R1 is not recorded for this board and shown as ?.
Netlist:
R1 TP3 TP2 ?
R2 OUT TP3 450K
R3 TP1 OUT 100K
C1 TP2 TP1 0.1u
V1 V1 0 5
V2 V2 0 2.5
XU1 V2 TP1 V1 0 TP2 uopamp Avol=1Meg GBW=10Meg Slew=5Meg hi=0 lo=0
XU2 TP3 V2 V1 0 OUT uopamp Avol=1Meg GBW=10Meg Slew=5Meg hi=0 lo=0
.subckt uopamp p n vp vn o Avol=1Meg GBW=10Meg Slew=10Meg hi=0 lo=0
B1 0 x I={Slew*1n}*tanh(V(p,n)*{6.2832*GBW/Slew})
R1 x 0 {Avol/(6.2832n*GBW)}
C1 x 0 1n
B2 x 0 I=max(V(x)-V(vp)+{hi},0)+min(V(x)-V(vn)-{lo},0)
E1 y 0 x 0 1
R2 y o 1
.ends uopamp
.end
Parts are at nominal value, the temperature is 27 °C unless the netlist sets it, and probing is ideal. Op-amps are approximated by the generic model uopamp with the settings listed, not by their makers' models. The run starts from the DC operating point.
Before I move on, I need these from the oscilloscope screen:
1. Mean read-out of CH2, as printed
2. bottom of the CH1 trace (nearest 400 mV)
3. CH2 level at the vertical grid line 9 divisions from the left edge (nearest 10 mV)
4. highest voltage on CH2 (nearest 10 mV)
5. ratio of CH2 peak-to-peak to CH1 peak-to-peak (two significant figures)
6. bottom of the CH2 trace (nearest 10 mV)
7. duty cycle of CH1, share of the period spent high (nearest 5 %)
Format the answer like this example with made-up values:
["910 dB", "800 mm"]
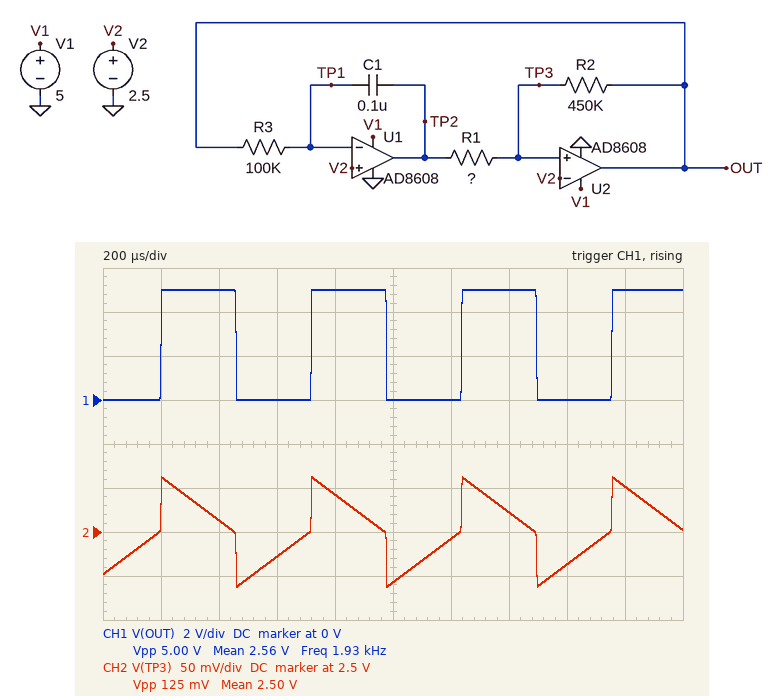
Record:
["2.50 V", "0 V", "2.55 V", "2.56 V", "0.025", "2.44 V", "50 %"]
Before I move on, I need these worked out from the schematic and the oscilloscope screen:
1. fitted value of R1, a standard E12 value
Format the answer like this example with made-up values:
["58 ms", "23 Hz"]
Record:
["5.6 kΩ"]
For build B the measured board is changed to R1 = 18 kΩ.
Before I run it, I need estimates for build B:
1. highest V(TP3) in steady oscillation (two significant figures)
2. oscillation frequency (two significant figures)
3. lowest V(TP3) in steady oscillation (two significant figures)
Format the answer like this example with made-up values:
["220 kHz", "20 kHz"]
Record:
["2.7 V", "620 Hz", "2.3 V"]
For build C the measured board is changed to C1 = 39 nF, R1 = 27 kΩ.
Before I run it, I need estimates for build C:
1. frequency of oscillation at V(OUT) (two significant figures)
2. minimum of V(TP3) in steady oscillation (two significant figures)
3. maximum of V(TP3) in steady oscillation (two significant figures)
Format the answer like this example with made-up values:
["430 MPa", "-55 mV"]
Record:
["1.1 kHz", "2.2 V", "2.8 V"]
